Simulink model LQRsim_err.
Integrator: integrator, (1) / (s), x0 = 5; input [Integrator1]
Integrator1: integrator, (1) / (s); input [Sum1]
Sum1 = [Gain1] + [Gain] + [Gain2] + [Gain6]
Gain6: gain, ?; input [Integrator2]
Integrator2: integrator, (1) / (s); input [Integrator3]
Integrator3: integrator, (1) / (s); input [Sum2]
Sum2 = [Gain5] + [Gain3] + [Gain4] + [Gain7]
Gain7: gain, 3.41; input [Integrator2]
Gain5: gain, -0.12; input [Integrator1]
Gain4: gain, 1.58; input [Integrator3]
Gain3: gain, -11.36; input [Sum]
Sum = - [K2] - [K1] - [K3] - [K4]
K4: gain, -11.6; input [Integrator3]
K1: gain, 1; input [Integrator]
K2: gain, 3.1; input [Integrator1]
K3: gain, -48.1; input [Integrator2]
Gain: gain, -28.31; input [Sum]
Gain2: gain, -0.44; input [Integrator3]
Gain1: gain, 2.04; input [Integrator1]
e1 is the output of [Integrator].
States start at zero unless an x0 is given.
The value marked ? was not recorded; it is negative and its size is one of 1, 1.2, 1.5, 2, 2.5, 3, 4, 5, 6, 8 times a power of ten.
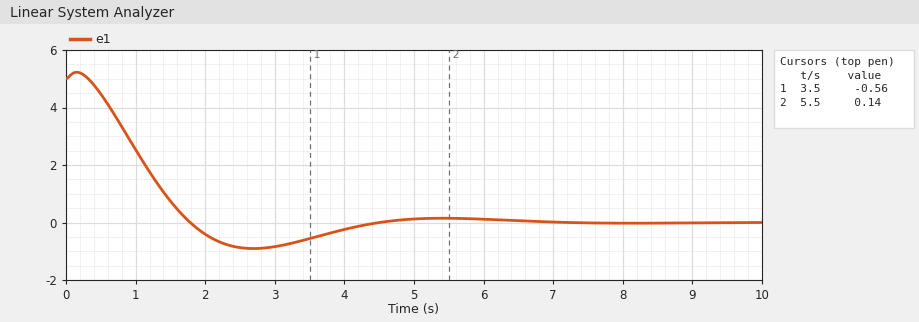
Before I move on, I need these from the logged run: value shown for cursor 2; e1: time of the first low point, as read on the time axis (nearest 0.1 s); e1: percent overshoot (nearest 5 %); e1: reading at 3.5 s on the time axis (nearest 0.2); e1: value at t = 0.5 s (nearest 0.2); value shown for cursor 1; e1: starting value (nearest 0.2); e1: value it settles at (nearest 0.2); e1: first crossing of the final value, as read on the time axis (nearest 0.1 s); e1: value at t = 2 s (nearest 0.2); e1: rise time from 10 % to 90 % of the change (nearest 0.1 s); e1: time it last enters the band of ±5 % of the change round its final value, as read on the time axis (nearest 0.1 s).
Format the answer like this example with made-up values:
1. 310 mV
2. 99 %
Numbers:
1. 0.14
2. 2.7 s
3. 20 %
4. -0.6
5. 4.4
6. -0.56
7. 5.0
8. 0.0
9. 1.8 s
10. -0.4
11. 1.1 s
12. 4.0 s
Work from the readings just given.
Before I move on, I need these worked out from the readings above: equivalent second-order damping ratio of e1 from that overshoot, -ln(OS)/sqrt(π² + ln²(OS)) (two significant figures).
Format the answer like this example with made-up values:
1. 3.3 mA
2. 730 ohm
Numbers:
1. 0.46
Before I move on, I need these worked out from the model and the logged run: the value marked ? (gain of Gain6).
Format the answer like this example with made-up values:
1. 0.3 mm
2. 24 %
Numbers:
1. -40
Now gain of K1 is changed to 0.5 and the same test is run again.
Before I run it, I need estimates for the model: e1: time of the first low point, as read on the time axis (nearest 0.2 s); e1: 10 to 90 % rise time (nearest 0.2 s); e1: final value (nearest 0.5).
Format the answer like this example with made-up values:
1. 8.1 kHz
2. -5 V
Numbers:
1. 4.8 s
2. 2.2 s
3. 0.0
